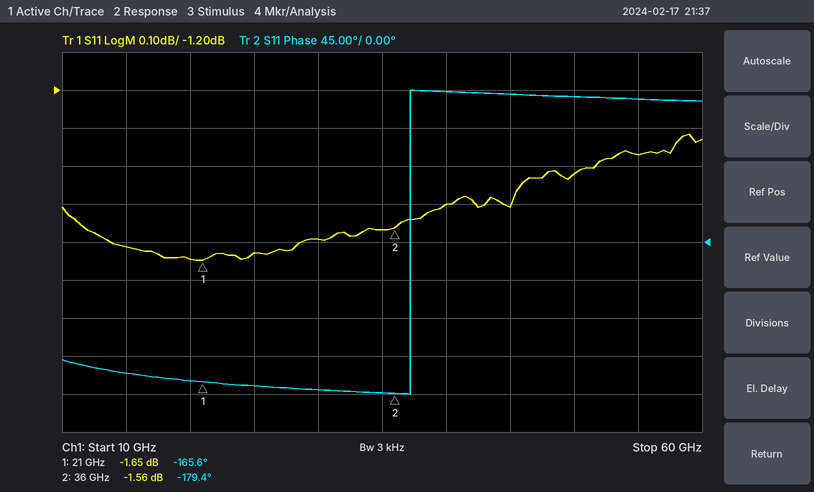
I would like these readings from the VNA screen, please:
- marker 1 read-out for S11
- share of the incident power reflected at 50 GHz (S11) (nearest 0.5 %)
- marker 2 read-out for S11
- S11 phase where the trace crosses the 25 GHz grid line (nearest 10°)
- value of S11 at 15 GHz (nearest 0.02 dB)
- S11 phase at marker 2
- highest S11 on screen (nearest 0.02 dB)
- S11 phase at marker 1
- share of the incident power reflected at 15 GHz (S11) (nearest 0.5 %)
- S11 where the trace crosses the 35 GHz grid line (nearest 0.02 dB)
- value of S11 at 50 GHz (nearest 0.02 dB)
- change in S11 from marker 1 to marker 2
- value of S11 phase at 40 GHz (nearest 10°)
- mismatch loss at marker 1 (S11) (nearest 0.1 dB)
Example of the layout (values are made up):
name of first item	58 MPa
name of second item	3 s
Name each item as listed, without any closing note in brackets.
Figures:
marker 1 read-out for S11	-1.65 dB
share of the incident power reflected at 50 GHz (S11)	72.0 %
marker 2 read-out for S11	-1.56 dB
S11 phase where the trace crosses the 25 GHz grid line	-170°
value of S11 at 15 GHz	-1.62 dB
S11 phase at marker 2	-179.4°
highest S11 on screen	-1.32 dB
S11 phase at marker 1	-165.6°
share of the incident power reflected at 15 GHz (S11)	69.0 %
S11 where the trace crosses the 35 GHz grid line	-1.56 dB
value of S11 at 50 GHz	-1.42 dB
change in S11 from marker 1 to marker 2	0.09 dB
value of S11 phase at 40 GHz	180°
mismatch loss at marker 1 (S11)	5.0 dB
